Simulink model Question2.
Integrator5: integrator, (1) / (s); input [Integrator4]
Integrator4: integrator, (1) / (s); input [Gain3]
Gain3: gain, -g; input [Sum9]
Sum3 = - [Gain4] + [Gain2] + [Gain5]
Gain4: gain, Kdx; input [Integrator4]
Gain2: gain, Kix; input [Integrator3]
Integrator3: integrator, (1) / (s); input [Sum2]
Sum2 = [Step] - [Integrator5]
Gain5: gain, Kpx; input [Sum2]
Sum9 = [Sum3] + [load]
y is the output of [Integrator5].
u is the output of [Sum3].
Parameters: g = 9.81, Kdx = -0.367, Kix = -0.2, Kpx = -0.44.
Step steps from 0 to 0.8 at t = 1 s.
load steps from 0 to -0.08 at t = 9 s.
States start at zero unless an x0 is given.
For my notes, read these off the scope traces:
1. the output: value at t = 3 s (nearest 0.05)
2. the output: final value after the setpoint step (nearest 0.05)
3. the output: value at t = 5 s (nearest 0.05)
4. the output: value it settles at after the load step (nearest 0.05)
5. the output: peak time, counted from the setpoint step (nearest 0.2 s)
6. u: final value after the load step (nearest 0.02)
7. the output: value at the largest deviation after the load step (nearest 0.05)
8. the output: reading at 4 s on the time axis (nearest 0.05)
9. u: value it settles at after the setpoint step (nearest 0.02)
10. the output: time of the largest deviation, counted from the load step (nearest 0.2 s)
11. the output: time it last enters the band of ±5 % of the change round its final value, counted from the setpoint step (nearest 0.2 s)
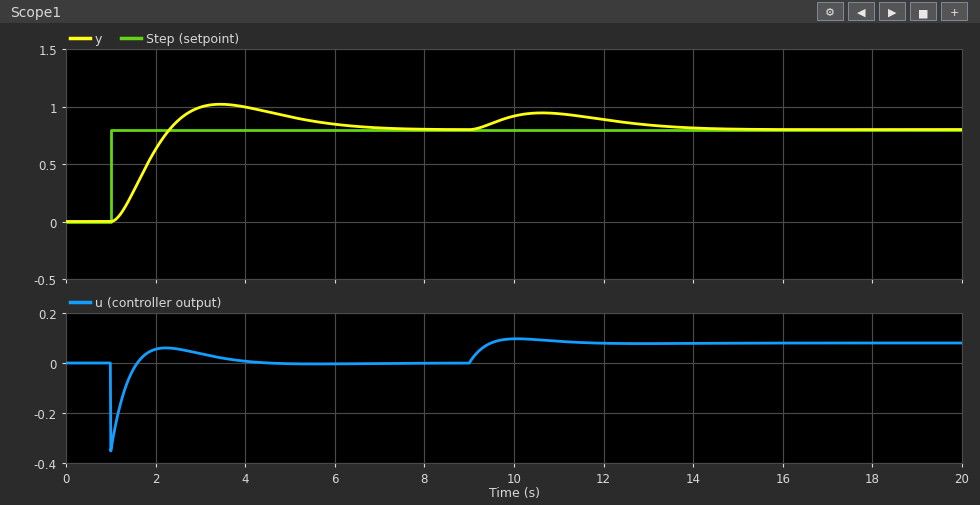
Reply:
1.00
0.80
0.90
0.80
2.4 s
0.08
0.95
1.00
0.00
1.6 s
5.2 s
